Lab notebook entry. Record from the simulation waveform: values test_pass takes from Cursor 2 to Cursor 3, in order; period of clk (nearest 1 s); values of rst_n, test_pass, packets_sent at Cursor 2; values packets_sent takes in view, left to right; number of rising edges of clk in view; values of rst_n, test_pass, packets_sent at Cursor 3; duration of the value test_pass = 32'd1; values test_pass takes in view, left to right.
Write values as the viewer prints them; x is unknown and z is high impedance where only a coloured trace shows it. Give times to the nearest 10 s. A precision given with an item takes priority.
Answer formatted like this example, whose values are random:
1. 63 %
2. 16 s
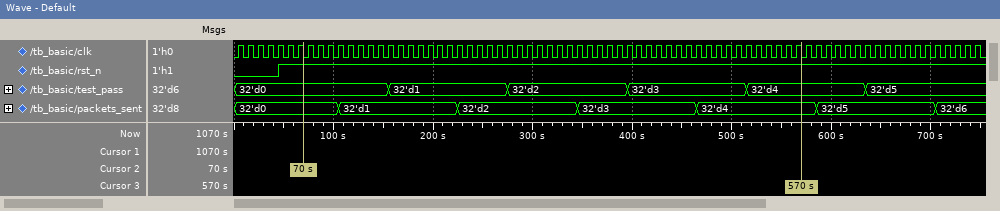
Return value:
1. 32'd0, 32'd1, 32'd2, 32'd3, 32'd4
2. 10 s
3. rst_n=1, test_pass=32'd0, packets_sent=32'd0
4. 32'd0, 32'd1, 32'd2, 32'd3, 32'd4, 32'd5, 32'd6
5. 75
6. rst_n=1, test_pass=32'd4, packets_sent=32'd4
7. 120 s
8. 32'd0, 32'd1, 32'd2, 32'd3, 32'd4, 32'd5
